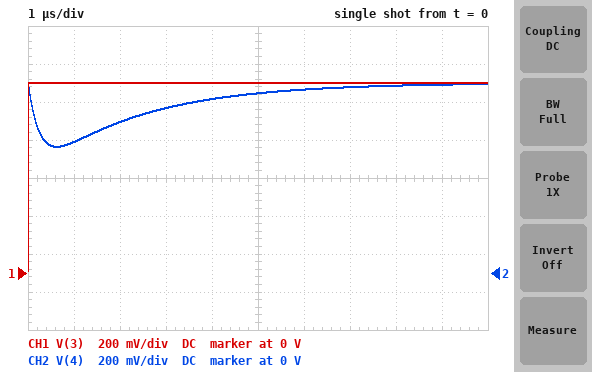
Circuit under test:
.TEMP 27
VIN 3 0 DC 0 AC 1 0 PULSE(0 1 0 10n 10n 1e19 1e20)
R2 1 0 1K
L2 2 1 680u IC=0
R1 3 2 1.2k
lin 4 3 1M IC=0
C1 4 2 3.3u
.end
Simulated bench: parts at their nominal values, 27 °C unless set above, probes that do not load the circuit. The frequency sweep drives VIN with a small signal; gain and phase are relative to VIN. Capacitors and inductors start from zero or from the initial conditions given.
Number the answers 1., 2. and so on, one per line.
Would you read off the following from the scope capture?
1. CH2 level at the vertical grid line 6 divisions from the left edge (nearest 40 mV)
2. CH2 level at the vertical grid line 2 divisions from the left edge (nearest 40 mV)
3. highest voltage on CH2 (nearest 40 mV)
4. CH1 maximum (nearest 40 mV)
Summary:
1. 960 mV
2. 800 mV
3. 1.00 V
4. 1.00 V
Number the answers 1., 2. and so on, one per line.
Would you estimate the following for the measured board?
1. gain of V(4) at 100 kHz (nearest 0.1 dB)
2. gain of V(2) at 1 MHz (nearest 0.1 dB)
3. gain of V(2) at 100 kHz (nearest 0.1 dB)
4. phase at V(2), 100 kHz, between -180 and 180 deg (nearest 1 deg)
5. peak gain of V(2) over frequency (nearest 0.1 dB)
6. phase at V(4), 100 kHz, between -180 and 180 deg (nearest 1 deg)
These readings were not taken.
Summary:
1. -3.1 dB
2. -1.1 dB
3. -3.1 dB
4. -13 deg
5. 0 dB
6. -13 deg
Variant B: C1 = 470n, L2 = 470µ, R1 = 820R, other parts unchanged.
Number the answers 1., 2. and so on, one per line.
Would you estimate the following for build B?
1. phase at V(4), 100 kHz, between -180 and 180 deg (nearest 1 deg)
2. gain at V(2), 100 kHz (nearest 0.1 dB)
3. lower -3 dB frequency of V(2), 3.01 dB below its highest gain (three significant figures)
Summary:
1. -12 deg
2. -3.0 dB
3. 471 Hz
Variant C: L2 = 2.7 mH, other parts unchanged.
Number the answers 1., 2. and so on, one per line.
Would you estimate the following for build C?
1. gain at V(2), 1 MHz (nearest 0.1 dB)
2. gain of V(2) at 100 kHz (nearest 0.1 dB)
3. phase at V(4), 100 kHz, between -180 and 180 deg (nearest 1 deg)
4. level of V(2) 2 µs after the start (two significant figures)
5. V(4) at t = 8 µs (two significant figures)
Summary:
1. -0.2 dB
2. -2.2 dB
3. -1 deg
4. 830 mV
5. 960 mV
